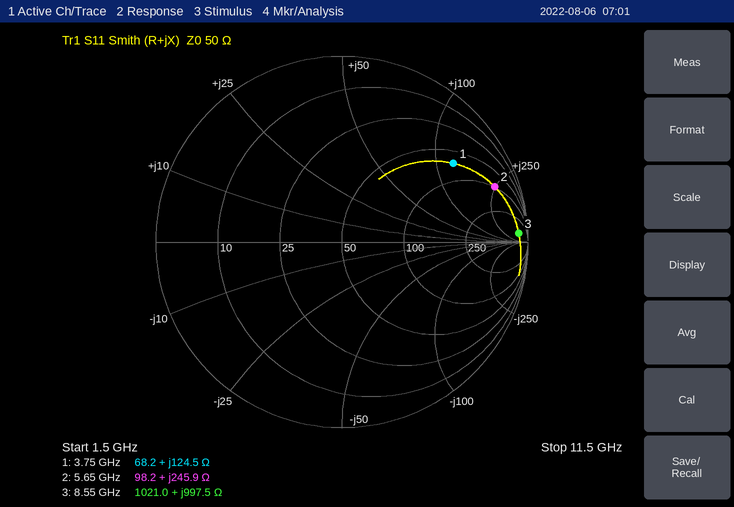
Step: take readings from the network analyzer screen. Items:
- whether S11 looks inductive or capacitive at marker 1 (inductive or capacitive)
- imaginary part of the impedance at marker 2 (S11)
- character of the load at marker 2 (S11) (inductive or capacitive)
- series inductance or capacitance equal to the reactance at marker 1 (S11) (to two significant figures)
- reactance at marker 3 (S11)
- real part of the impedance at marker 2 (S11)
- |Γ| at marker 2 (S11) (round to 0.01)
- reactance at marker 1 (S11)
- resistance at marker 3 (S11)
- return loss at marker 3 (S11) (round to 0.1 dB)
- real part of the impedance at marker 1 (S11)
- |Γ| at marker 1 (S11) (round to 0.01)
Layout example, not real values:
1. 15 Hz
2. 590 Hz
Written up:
1. inductive
2. +245.9 Ω
3. inductive
4. 5.3 nH
5. +997.5 Ω
6. 98.2 Ω
7. 0.87
8. +124.5 Ω
9. 1021.0 Ω
10. 0.4 dB
11. 68.2 Ω
12. 0.73
